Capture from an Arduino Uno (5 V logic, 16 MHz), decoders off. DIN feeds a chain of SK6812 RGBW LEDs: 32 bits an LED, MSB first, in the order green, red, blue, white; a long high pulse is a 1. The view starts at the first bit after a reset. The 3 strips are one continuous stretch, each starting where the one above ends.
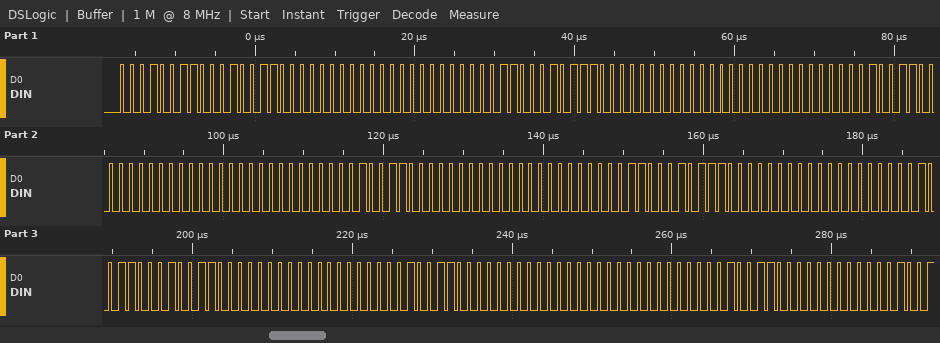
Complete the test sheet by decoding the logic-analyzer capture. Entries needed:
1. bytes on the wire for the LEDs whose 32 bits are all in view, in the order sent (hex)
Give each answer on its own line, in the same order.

13 13 00 00 03 17 00 00 00 13 00 00 00 13 00 00 03 17 00 00 13 13 00 00 13 00 00 00
